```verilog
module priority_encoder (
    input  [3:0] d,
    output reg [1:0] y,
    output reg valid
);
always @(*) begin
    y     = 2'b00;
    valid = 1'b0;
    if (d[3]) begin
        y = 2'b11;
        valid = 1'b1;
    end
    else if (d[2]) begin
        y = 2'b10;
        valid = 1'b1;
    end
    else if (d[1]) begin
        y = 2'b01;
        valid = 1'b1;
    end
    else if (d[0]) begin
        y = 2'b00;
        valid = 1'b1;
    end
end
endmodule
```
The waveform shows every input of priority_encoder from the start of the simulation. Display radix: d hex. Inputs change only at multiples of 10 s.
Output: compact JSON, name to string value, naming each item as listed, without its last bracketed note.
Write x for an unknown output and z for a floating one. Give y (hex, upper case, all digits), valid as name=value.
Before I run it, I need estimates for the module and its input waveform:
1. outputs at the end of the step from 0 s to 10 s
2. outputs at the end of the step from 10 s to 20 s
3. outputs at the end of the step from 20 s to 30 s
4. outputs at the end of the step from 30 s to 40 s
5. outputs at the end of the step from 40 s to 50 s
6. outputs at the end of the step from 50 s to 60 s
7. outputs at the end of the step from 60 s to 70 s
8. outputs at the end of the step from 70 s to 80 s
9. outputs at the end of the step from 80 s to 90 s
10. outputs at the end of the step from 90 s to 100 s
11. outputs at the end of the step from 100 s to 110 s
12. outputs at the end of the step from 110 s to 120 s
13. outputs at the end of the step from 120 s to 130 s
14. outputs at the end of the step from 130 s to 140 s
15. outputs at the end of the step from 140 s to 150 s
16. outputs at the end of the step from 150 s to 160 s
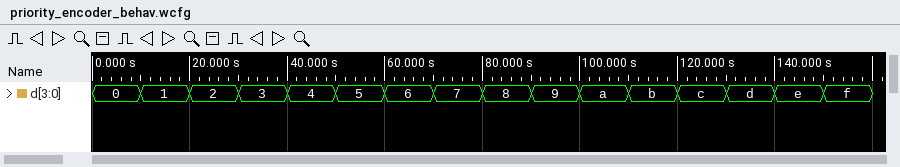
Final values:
{"outputs at the end of the step from 0 s to 10 s": "y=0, valid=0", "outputs at the end of the step from 10 s to 20 s": "y=0, valid=1", "outputs at the end of the step from 20 s to 30 s": "y=1, valid=1", "outputs at the end of the step from 30 s to 40 s": "y=1, valid=1", "outputs at the end of the step from 40 s to 50 s": "y=2, valid=1", "outputs at the end of the step from 50 s to 60 s": "y=2, valid=1", "outputs at the end of the step from 60 s to 70 s": "y=2, valid=1", "outputs at the end of the step from 70 s to 80 s": "y=2, valid=1", "outputs at the end of the step from 80 s to 90 s": "y=3, valid=1", "outputs at the end of the step from 90 s to 100 s": "y=3, valid=1", "outputs at the end of the step from 100 s to 110 s": "y=3, valid=1", "outputs at the end of the step from 110 s to 120 s": "y=3, valid=1", "outputs at the end of the step from 120 s to 130 s": "y=3, valid=1", "outputs at the end of the step from 130 s to 140 s": "y=3, valid=1", "outputs at the end of the step from 140 s to 150 s": "y=3, valid=1", "outputs at the end of the step from 150 s to 160 s": "y=3, valid=1"}
